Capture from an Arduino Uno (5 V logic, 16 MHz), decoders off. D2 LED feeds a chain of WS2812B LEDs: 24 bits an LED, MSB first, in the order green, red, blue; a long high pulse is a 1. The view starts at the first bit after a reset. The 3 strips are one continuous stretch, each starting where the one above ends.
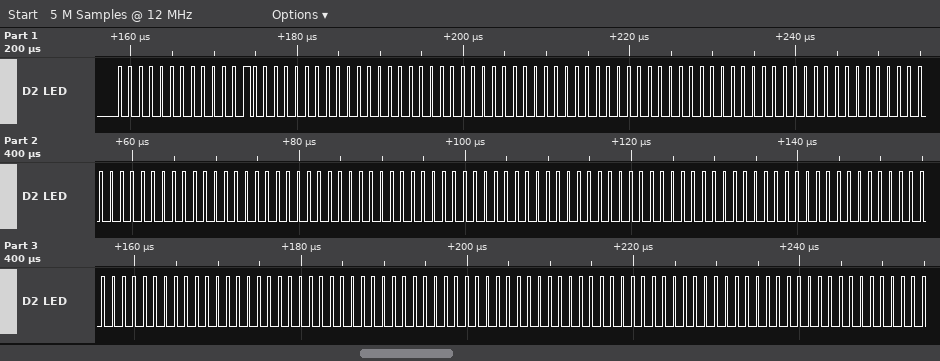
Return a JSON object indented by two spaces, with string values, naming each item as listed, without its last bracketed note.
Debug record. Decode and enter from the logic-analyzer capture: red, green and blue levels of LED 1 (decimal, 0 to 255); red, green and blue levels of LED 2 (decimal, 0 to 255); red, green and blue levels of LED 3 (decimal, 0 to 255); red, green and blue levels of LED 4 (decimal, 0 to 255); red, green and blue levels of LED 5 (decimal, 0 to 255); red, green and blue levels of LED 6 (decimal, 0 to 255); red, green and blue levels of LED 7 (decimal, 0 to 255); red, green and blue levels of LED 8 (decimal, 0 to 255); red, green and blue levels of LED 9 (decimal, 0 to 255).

{
  "red, green and blue levels of LED 1": "8, 0, 0",
  "red, green and blue levels of LED 2": "0, 0, 0",
  "red, green and blue levels of LED 3": "0, 0, 0",
  "red, green and blue levels of LED 4": "0, 0, 0",
  "red, green and blue levels of LED 5": "0, 0, 0",
  "red, green and blue levels of LED 6": "0, 0, 0",
  "red, green and blue levels of LED 7": "0, 0, 0",
  "red, green and blue levels of LED 8": "0, 0, 0",
  "red, green and blue levels of LED 9": "0, 0, 0"
}
